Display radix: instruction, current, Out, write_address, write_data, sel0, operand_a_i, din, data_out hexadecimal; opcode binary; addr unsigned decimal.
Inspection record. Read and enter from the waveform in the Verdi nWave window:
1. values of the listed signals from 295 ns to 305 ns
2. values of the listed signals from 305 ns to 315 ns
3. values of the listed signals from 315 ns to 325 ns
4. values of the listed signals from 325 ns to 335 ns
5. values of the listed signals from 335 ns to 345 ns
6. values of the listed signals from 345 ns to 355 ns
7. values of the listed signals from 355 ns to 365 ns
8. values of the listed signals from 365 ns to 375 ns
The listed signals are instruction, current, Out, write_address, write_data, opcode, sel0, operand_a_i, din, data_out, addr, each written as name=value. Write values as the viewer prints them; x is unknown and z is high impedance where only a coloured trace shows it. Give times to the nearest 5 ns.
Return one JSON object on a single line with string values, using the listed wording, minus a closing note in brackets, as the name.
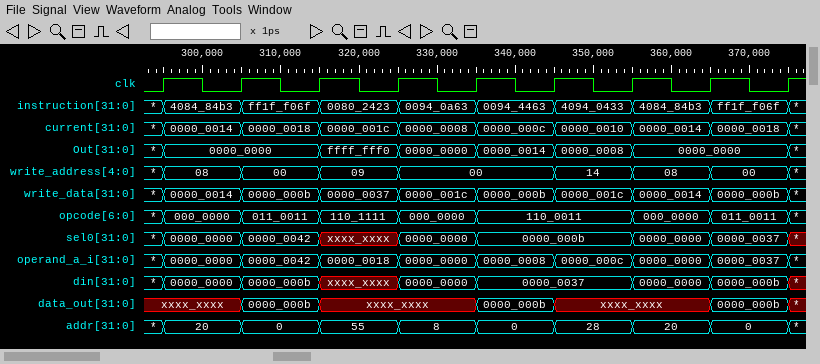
{"values of the listed signals from 295 ns to 305 ns": "instruction=4084_84b3, current=0000_0014, Out=0000_0000, write_address=08, write_data=0000_0014, opcode=000_0000, sel0=0000_0000, operand_a_i=0000_0000, din=0000_0000, data_out=xxxx_xxxx, addr=20", "values of the listed signals from 305 ns to 315 ns": "instruction=ff1f_f06f, current=0000_0018, Out=0000_0000, write_address=00, write_data=0000_000b, opcode=011_0011, sel0=0000_0042, operand_a_i=0000_0042, din=0000_000b, data_out=0000_000b, addr=0", "values of the listed signals from 315 ns to 325 ns": "instruction=0080_2423, current=0000_001c, Out=ffff_fff0, write_address=09, write_data=0000_0037, opcode=110_1111, sel0=xxxx_xxxx, operand_a_i=0000_0018, din=xxxx_xxxx, data_out=xxxx_xxxx, addr=55", "values of the listed signals from 325 ns to 335 ns": "instruction=0094_0a63, current=0000_0008, Out=0000_0000, write_address=00, write_data=0000_001c, opcode=000_0000, sel0=0000_0000, operand_a_i=0000_0000, din=0000_0000, data_out=xxxx_xxxx, addr=8", "values of the listed signals from 335 ns to 345 ns": "instruction=0094_4463, current=0000_000c, Out=0000_0014, write_address=00, write_data=0000_000b, opcode=110_0011, sel0=0000_000b, operand_a_i=0000_0008, din=0000_0037, data_out=0000_000b, addr=0", "values of the listed signals from 345 ns to 355 ns": "instruction=4094_0433, current=0000_0010, Out=0000_0008, write_address=14, write_data=0000_001c, opcode=110_0011, sel0=0000_000b, operand_a_i=0000_000c, din=0000_0037, data_out=xxxx_xxxx, addr=28", "values of the listed signals from 355 ns to 365 ns": "instruction=4084_84b3, current=0000_0014, Out=0000_0000, write_address=08, write_data=0000_0014, opcode=000_0000, sel0=0000_0000, operand_a_i=0000_0000, din=0000_0000, data_out=xxxx_xxxx, addr=20", "values of the listed signals from 365 ns to 375 ns": "instruction=ff1f_f06f, current=0000_0018, Out=0000_0000, write_address=00, write_data=0000_000b, opcode=011_0011, sel0=0000_0037, operand_a_i=0000_0037, din=0000_000b, data_out=0000_000b, addr=0"}
